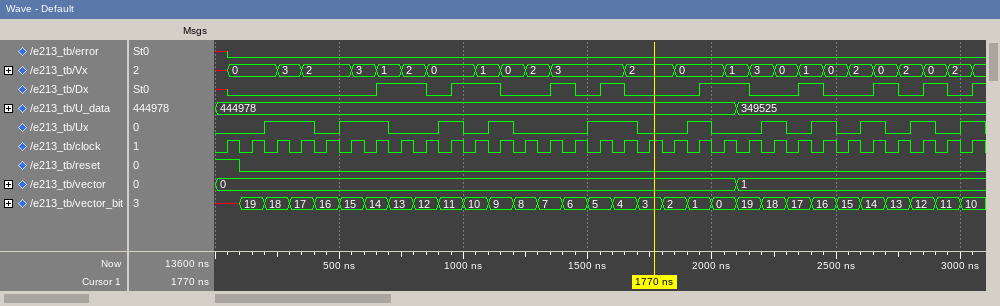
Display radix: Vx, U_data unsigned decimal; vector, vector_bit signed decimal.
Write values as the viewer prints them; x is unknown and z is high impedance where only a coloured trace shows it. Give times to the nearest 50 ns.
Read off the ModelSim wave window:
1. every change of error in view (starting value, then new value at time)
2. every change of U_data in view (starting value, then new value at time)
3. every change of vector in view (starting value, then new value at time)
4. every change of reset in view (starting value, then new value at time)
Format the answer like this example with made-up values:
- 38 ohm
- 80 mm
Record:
- x, 0 at 50 ns
- 444978, 349525 at 2100 ns
- 0, 1 at 2100 ns
- 1, 0 at 100 ns
